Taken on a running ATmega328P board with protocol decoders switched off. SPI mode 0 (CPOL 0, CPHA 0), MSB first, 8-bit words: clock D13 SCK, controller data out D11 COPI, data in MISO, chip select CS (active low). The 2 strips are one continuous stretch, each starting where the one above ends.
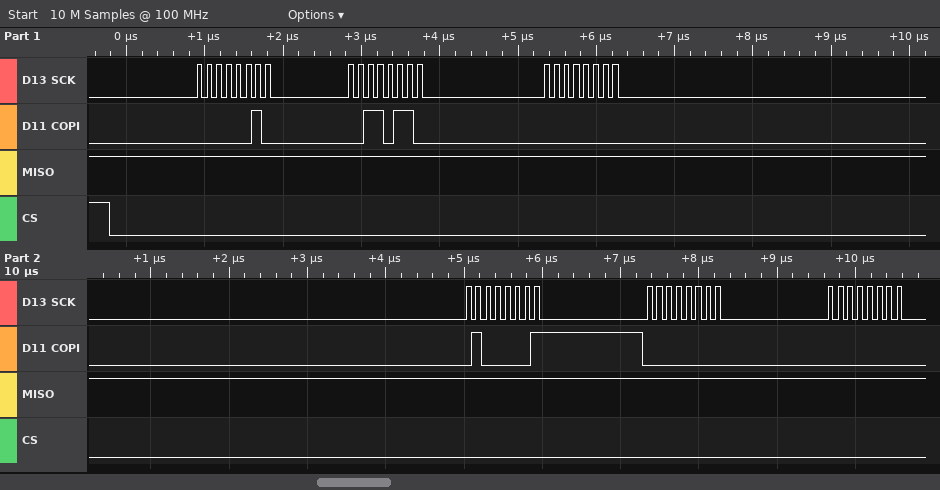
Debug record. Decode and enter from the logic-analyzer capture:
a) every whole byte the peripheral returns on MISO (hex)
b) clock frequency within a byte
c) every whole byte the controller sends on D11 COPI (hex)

0xFF 0xFF 0xFF 0xFF 0xFF 0xFF
8 MHz
0x02 0x36 0x00 0x41 0x00 0x00
